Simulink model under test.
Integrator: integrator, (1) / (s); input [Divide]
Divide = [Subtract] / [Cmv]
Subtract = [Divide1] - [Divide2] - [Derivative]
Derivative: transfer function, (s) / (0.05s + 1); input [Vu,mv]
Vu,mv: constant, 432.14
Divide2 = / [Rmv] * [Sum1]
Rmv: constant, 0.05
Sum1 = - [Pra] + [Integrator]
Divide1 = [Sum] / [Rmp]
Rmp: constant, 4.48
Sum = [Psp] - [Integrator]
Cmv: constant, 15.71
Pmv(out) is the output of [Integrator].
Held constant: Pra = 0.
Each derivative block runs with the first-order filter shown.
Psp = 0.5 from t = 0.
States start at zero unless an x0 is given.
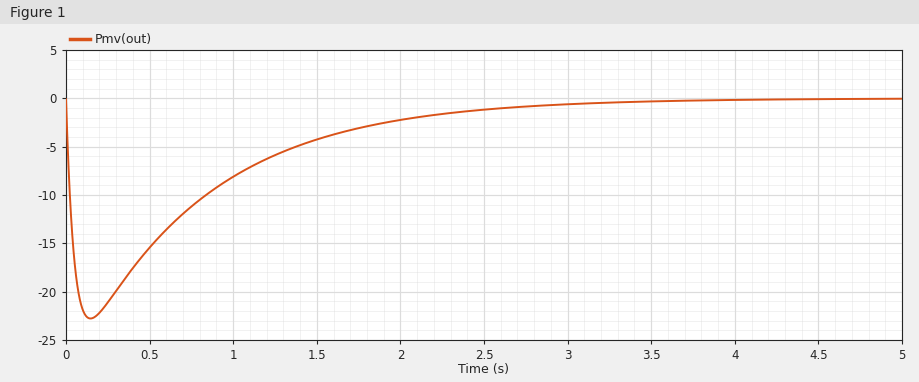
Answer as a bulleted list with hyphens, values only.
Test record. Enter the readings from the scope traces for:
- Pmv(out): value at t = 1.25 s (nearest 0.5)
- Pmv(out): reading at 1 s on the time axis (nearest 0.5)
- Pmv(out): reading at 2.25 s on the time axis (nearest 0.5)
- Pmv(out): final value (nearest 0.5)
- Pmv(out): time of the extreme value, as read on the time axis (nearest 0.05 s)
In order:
- -6.0
- -8.0
- -1.5
- 0.0
- 0.15 s
